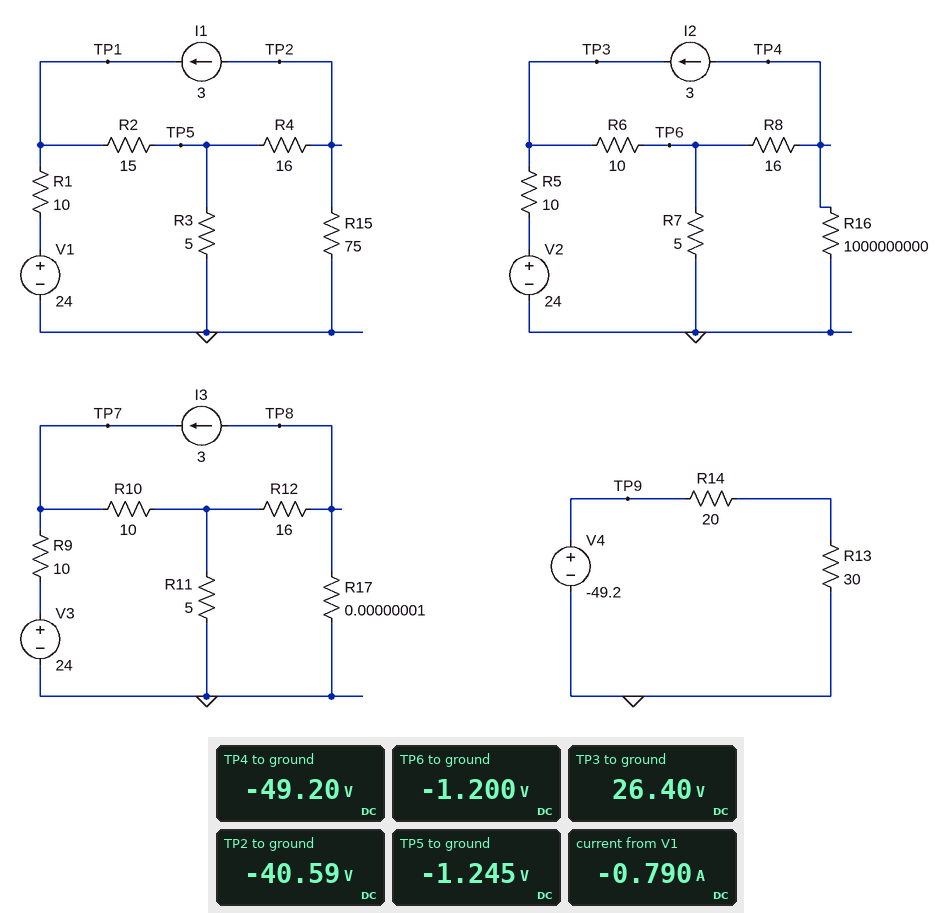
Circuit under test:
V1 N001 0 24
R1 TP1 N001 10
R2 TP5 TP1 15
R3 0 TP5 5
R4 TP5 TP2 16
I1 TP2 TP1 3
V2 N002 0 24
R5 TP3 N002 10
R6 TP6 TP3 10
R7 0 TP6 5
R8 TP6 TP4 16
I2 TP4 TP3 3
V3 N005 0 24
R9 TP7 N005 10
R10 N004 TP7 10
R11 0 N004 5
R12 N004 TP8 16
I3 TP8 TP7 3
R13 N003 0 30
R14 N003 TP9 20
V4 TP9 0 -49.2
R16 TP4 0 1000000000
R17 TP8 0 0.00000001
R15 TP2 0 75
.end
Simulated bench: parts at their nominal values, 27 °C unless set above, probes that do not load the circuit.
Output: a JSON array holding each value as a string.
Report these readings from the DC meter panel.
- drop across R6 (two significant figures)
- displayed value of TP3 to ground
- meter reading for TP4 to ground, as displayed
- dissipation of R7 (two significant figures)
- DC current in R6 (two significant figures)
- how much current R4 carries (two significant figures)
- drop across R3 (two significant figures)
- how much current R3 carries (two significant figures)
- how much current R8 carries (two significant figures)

["28 V", "26.40 V", "-49.20 V", "290 mW", "2.8 A", "2.5 A", "1.2 V", "250 mA", "3.0 A"]
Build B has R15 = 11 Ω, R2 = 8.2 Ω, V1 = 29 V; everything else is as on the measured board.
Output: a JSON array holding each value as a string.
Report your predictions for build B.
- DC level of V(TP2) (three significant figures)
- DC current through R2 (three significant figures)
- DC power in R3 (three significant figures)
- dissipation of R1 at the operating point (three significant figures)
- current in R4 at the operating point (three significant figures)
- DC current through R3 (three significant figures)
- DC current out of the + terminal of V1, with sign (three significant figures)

["-16.7 V", "2.86 A", "9.57 W", "191 mW", "1.48 A", "1.38 A", "-138 mA"]
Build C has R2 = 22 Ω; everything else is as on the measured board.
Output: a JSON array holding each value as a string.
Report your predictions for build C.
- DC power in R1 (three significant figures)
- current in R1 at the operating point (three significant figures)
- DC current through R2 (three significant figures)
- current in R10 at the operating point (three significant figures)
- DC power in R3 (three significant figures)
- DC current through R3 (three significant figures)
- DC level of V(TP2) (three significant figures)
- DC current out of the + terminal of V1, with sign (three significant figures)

["14.7 W", "1.21 A", "1.79 A", "2.27 A", "2.10 W", "648 mA", "-42.2 V", "-1.21 A"]
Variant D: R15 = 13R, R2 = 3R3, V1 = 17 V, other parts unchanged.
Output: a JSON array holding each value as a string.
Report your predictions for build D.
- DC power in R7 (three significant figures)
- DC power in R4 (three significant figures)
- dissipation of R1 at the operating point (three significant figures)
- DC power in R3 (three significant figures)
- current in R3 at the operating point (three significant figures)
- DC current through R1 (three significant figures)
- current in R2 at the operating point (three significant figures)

["288 mW", "40.4 W", "55.0 µW", "9.99 W", "1.41 A", "2.34 mA", "3.00 A"]
